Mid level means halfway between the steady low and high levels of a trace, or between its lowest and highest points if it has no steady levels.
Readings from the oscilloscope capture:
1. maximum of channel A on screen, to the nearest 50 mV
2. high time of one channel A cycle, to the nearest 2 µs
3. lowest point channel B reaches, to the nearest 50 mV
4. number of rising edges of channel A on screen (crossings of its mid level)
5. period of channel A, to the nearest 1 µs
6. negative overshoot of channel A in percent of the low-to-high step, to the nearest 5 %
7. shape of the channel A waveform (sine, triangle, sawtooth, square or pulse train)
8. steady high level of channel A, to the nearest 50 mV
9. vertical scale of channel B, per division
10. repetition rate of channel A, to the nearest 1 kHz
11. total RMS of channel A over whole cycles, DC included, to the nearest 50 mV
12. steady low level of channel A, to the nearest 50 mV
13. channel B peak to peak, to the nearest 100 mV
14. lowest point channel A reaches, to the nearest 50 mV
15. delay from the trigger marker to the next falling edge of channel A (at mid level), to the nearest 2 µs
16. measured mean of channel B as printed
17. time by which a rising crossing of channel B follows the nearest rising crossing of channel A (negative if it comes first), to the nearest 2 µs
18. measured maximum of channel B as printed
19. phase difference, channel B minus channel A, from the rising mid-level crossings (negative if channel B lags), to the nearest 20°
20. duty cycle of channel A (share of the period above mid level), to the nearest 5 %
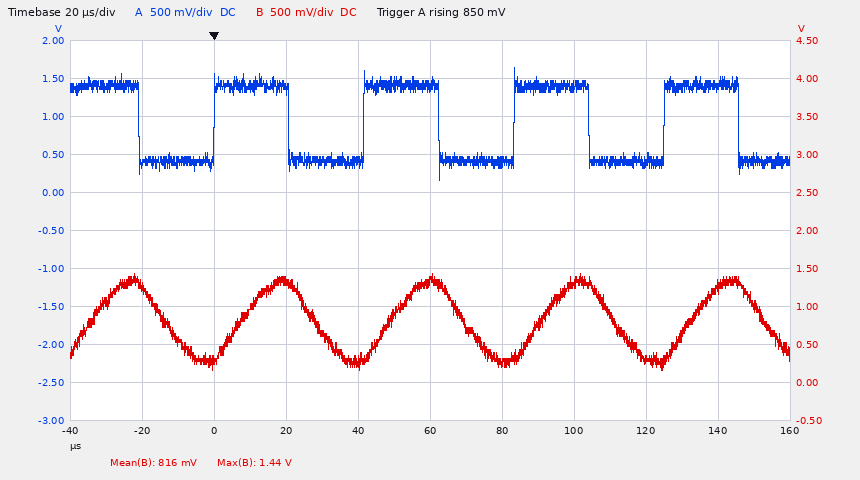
1.65 V
20 µs
150 mV
4
42 µs
25 %
square
1.40 V
500 mV
24 kHz
1.05 V
400 mV
1.30 V
150 mV
20 µs
816 mV
+8 µs
1.44 V
-60°
50 %
